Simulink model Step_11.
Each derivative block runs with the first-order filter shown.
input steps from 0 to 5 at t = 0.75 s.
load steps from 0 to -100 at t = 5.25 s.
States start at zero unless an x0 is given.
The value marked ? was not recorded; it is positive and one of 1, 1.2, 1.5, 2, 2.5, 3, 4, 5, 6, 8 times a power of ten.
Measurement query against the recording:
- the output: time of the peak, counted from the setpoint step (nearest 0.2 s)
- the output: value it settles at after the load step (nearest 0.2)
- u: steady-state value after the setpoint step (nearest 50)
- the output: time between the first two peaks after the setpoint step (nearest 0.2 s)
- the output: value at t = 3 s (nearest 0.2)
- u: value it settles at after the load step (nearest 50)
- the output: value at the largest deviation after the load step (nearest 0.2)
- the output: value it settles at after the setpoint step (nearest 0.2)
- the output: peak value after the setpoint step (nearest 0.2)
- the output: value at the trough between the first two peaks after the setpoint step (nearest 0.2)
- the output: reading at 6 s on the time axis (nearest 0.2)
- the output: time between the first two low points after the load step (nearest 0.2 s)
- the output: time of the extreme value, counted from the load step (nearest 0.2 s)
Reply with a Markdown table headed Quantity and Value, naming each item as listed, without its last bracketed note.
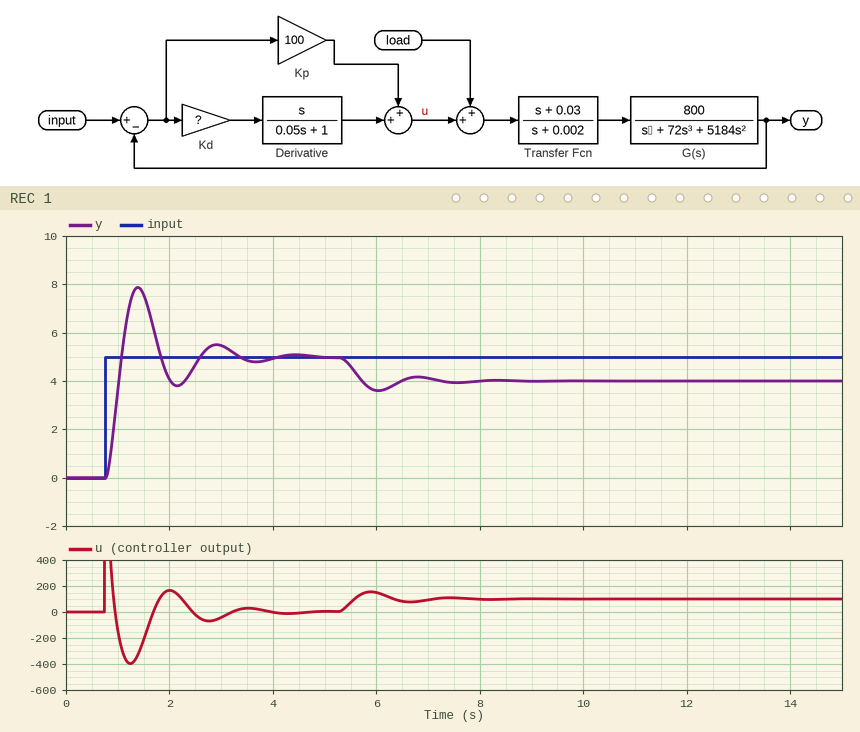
| Quantity | Value |
|---|---|
| the output: time of the peak, counted from the setpoint step | 0.6 s |
| the output: value it settles at after the load step | 4.0 |
| u: steady-state value after the setpoint step | 0 |
| the output: time between the first two peaks after the setpoint step | 1.6 s |
| the output: value at t = 3 s | 5.4 |
| u: value it settles at after the load step | 100 |
| the output: value at the largest deviation after the load step | 3.6 |
| the output: value it settles at after the setpoint step | 5.0 |
| the output: peak value after the setpoint step | 7.8 |
| the output: value at the trough between the first two peaks after the setpoint step | 3.8 |
| the output: reading at 6 s on the time axis | 3.6 |
| the output: time between the first two low points after the load step | 1.6 s |
| the output: time of the extreme value, counted from the load step | 0.8 s |
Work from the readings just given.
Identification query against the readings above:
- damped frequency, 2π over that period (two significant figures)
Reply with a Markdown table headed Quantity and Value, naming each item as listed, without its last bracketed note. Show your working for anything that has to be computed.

| Quantity | Value |
|---|---|
| damped frequency, 2π over that period | 2π / 1.6 = 3.9 rad/s |
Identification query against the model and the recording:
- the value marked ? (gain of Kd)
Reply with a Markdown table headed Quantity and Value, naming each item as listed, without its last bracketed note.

| Quantity | Value |
|---|---|
| the value marked ? | 15 |
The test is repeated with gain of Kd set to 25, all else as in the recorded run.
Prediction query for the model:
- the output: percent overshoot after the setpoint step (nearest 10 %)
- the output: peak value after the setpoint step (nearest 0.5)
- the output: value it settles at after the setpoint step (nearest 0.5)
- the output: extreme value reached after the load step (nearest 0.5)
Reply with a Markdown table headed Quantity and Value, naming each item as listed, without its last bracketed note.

| Quantity | Value |
|---|---|
| the output: percent overshoot after the setpoint step | 40 % |
| the output: peak value after the setpoint step | 7.0 |
| the output: value it settles at after the setpoint step | 5.0 |
| the output: extreme value reached after the load step | 4.0 |
